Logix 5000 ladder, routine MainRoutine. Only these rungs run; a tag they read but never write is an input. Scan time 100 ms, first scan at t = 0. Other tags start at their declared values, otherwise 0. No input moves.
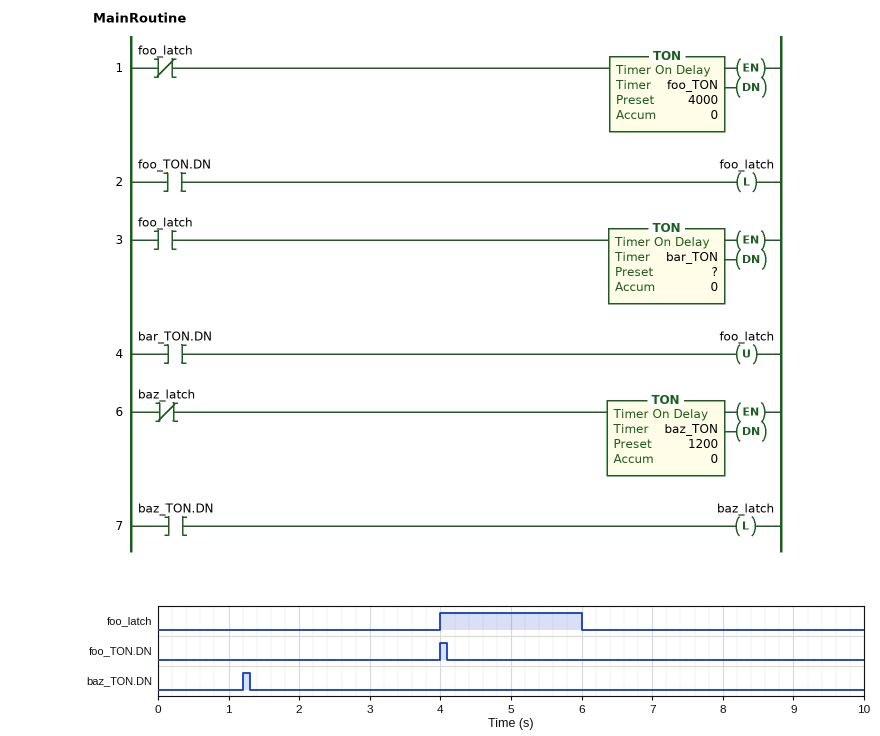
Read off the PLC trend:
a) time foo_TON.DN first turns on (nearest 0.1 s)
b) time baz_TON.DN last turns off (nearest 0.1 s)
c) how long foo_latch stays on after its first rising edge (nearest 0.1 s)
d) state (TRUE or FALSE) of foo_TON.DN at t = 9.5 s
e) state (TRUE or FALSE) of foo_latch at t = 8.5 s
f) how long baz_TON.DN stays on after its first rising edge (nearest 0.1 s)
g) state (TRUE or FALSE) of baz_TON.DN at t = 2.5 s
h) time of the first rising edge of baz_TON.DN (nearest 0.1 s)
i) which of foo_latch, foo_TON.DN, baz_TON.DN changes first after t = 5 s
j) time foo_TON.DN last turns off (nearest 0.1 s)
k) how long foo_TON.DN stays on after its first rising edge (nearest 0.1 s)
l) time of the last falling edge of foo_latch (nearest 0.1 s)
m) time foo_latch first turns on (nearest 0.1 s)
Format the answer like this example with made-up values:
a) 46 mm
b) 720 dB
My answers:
a) 4.0 s
b) 1.3 s
c) 2.0 s
d) FALSE
e) FALSE
f) 0.1 s
g) FALSE
h) 1.2 s
i) foo_latch
j) 4.1 s
k) 0.1 s
l) 6.0 s
m) 4.0 s
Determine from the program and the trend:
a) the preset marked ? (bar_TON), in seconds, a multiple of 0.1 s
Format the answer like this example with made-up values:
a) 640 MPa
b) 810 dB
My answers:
a) 2.0 s
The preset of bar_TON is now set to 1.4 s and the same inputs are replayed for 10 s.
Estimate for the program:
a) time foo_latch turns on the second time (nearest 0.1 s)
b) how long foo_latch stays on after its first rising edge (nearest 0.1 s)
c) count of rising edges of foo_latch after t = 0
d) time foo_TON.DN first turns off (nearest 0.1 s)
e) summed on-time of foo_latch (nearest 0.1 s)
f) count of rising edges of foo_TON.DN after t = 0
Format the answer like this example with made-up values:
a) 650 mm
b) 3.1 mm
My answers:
a) 9.5 s
b) 1.4 s
c) 2
d) 4.1 s
e) 1.9 s
f) 2
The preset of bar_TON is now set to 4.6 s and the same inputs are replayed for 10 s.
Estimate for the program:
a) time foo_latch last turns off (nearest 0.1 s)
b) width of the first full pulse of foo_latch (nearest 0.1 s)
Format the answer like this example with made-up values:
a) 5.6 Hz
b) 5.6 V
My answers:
a) 8.6 s
b) 4.6 s
